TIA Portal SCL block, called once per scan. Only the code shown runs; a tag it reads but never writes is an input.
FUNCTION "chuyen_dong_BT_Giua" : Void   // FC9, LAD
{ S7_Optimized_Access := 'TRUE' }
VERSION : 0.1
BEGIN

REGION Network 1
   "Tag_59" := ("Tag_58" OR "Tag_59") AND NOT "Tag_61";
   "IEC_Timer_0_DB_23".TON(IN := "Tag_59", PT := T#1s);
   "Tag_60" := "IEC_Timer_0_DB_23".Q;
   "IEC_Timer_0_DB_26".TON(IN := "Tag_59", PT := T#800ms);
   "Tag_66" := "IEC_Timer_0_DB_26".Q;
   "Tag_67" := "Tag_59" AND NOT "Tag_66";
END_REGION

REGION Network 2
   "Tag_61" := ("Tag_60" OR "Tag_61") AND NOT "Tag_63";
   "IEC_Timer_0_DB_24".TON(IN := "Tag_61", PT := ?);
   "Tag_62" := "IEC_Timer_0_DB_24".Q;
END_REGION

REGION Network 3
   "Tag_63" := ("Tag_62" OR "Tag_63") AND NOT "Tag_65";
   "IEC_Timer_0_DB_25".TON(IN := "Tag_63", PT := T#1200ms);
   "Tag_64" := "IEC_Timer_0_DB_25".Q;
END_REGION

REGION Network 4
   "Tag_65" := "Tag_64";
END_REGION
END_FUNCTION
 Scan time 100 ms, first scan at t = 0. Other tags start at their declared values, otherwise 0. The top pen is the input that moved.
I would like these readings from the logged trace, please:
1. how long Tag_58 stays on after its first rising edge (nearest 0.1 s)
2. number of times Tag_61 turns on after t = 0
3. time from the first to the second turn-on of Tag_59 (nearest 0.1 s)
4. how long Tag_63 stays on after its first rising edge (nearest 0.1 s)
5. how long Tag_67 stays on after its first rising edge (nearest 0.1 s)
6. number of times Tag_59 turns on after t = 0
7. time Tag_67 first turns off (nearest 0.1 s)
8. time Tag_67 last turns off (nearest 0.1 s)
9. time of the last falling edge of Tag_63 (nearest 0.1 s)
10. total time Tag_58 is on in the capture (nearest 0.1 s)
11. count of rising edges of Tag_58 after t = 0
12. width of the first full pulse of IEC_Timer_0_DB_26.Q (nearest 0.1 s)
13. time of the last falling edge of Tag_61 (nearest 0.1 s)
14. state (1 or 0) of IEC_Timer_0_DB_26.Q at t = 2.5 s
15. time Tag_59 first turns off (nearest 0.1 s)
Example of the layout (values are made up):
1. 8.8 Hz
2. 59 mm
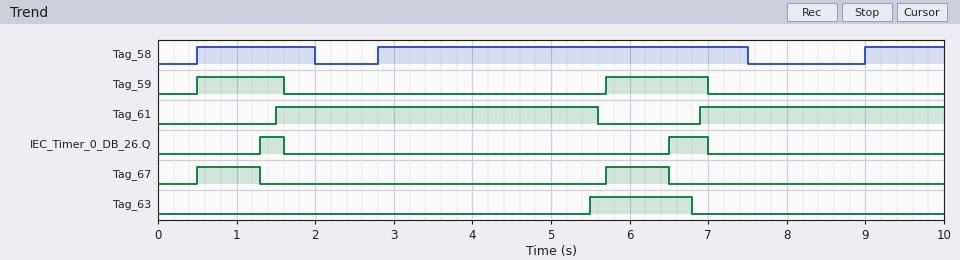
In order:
1. 1.5 s
2. 2
3. 5.2 s
4. 1.3 s
5. 0.8 s
6. 2
7. 1.3 s
8. 6.5 s
9. 6.8 s
10. 7.2 s
11. 3
12. 0.3 s
13. 5.6 s
14. 0
15. 1.6 s
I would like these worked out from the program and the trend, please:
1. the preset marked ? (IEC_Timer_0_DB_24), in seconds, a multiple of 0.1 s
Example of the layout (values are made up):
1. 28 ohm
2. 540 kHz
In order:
1. 4.0 s
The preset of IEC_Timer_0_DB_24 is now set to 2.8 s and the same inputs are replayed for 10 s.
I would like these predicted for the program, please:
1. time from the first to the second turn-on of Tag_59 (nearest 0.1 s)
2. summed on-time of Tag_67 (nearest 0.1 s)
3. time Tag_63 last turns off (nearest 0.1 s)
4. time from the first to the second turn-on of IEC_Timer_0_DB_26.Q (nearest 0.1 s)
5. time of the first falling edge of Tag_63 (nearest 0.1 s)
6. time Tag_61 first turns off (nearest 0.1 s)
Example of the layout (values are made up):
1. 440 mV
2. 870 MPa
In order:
1. 4.0 s
2. 2.4 s
3. 9.8 s
4. 4.0 s
5. 5.6 s
6. 4.4 s
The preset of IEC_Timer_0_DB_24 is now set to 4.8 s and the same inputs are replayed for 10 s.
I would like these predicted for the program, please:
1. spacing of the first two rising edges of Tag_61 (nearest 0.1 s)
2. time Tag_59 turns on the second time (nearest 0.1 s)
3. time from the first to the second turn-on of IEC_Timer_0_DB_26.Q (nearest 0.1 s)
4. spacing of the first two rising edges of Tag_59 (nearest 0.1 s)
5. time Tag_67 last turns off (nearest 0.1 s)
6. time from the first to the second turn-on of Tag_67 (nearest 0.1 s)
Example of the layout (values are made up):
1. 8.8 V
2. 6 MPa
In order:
1. 6.2 s
2. 6.5 s
3. 6.0 s
4. 6.0 s
5. 7.3 s
6. 6.0 s
